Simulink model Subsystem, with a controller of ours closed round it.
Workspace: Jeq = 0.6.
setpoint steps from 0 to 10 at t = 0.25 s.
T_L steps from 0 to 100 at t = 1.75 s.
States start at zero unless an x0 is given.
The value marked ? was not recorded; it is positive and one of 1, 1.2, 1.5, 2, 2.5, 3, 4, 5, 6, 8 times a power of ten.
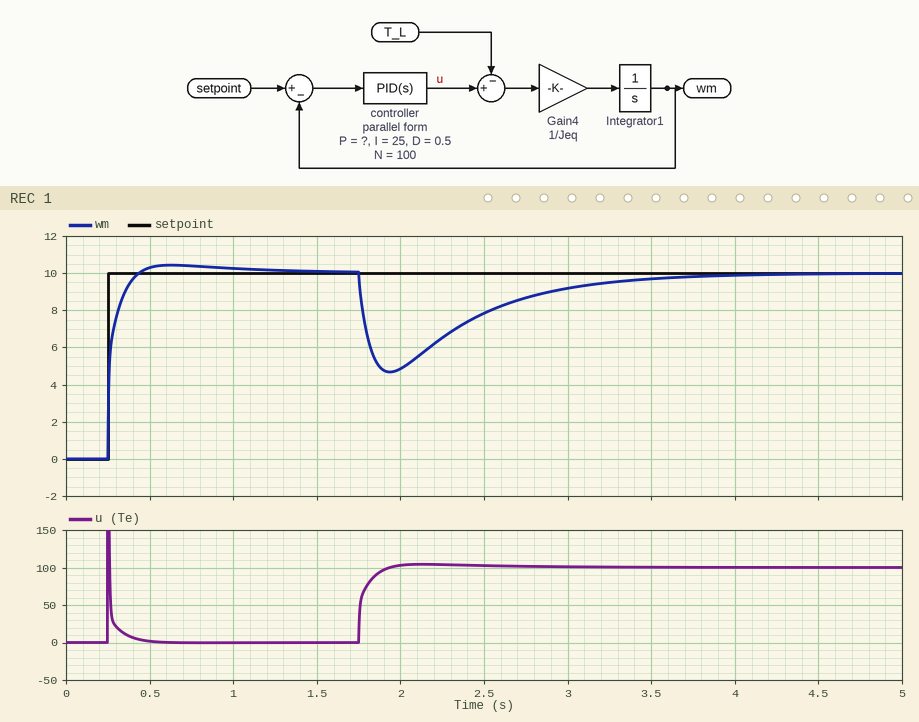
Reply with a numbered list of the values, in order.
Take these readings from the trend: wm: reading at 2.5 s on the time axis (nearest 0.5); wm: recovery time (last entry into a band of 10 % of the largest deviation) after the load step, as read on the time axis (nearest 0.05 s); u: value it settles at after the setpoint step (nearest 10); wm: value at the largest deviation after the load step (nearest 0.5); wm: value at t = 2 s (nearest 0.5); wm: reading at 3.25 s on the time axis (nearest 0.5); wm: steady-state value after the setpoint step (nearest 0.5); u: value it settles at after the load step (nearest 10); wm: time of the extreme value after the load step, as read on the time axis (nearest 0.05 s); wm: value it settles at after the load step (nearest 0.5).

1. 8.0
2. 3.20 s
3. 0
4. 4.5
5. 5.0
6. 9.5
7. 10.0
8. 100
9. 1.95 s
10. 10.0
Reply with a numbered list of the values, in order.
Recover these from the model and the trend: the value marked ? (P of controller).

1. 15
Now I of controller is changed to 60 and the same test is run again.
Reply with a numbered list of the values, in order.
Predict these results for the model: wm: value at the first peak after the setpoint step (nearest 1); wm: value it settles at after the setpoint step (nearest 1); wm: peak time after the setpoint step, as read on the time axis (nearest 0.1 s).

1. 11
2. 10
3. 0.5 s
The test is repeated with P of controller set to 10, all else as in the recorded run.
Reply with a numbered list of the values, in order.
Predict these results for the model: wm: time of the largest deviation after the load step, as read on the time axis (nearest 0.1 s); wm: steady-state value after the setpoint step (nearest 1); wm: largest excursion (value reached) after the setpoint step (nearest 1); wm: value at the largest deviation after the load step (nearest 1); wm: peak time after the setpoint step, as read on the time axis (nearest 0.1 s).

1. 2.0 s
2. 10
3. 11
4. 3
5. 0.7 s
